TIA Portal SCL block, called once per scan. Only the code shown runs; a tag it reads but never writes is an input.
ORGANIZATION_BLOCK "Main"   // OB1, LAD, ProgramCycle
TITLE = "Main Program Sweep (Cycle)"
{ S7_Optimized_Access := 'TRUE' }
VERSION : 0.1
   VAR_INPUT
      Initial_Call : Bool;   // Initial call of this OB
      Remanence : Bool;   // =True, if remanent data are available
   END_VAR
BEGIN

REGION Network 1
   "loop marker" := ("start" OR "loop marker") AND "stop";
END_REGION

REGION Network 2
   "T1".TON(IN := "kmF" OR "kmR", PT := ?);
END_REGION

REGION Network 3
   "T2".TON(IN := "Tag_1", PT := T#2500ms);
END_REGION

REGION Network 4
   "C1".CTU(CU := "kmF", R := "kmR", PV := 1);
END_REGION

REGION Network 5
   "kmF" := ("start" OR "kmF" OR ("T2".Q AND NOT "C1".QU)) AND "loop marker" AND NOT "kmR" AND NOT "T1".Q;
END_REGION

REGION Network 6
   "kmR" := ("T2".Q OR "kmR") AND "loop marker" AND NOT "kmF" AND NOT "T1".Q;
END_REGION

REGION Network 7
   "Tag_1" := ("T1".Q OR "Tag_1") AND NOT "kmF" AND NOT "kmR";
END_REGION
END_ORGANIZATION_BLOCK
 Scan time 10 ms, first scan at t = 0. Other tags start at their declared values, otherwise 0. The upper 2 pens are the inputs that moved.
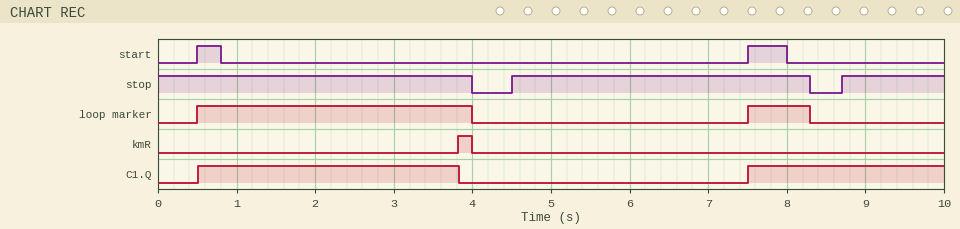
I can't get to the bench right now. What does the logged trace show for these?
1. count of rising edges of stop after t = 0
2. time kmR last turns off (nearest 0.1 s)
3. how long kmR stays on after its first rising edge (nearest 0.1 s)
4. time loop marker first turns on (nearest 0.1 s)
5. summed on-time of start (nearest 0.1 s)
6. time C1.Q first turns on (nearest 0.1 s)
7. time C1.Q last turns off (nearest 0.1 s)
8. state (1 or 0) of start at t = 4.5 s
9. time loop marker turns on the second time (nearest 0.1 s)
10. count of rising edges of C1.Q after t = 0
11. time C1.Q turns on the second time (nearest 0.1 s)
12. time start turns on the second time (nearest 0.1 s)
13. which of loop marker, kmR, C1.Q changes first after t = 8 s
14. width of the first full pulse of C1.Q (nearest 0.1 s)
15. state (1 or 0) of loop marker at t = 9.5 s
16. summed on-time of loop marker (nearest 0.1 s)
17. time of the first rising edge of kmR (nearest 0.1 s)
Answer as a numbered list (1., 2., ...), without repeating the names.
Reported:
1. 2
2. 4.0 s
3. 0.2 s
4. 0.5 s
5. 0.8 s
6. 0.5 s
7. 3.8 s
8. 0
9. 7.5 s
10. 2
11. 7.5 s
12. 7.5 s
13. loop marker
14. 3.3 s
15. 0
16. 4.3 s
17. 3.8 s
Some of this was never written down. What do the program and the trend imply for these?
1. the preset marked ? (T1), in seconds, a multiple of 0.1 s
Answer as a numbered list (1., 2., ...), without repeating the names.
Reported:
1. 0.8 s
